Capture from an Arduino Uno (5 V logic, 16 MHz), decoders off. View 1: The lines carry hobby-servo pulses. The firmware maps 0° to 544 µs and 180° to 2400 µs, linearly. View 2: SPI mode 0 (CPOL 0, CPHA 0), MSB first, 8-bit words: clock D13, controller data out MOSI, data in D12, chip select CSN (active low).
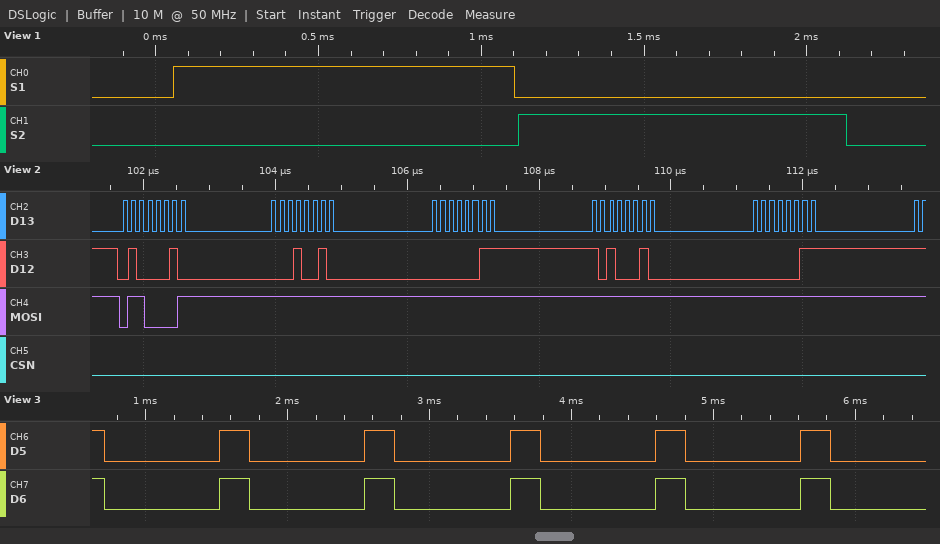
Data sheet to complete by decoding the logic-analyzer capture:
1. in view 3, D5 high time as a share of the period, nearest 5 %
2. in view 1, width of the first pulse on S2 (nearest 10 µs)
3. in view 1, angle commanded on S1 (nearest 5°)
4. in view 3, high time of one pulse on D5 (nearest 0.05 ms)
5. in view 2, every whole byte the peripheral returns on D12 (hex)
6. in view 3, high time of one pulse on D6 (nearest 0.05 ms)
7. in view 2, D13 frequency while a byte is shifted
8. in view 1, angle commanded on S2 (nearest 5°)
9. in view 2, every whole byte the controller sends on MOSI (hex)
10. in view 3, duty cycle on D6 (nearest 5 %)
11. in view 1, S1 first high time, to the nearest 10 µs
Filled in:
20 %
1010 µs
50°
0.20 ms
42 12 03 A2 03
0.20 ms
8 MHz
45°
61 FF FF FF FF
20 %
1050 µs
